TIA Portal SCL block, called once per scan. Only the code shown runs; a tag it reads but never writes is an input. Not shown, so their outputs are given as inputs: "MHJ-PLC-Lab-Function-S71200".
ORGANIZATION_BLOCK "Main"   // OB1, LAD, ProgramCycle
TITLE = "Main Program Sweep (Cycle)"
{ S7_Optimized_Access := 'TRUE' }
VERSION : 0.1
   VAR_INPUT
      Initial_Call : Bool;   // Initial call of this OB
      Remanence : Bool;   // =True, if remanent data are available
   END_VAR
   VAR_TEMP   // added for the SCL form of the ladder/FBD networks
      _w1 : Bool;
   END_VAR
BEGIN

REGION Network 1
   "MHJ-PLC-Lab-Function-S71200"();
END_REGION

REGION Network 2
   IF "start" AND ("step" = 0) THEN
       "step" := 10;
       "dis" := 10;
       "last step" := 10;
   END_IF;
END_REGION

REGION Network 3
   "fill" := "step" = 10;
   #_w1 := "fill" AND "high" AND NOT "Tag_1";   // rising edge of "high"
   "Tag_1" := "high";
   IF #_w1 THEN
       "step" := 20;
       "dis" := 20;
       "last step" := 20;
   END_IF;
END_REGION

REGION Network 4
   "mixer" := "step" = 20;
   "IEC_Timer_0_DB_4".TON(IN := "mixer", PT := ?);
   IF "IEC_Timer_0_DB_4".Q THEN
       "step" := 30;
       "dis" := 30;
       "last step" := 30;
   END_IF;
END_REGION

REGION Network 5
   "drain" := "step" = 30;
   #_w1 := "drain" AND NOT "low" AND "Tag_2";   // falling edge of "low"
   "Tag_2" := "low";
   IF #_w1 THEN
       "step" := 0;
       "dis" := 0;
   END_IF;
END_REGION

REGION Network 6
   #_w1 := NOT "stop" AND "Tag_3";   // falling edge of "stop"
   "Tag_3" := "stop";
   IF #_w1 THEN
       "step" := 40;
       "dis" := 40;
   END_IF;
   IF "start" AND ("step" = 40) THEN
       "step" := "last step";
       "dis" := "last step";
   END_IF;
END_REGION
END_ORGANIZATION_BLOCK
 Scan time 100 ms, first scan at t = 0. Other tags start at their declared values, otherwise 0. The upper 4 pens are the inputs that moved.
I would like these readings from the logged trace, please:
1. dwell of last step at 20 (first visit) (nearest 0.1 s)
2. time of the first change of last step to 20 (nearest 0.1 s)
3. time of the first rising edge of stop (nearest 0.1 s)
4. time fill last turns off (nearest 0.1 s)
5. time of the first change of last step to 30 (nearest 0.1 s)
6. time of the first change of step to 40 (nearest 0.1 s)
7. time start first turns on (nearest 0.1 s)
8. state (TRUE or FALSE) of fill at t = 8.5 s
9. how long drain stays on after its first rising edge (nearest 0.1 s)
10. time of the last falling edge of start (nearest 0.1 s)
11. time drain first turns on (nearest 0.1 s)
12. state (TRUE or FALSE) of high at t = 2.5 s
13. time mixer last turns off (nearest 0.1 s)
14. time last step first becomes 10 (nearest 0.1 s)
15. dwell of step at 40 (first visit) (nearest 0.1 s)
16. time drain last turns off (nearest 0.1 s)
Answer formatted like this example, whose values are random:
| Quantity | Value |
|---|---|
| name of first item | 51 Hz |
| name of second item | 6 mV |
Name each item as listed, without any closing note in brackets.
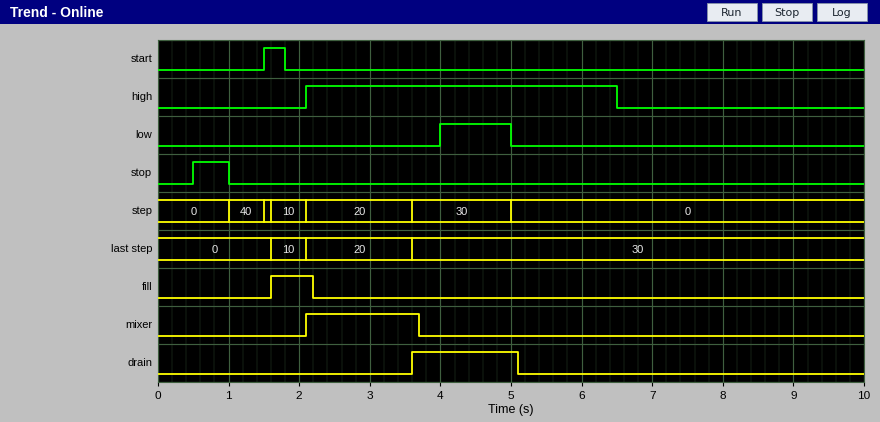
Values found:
| Quantity | Value |
|---|---|
| dwell of last step at 20 (first visit) | 1.5 s |
| time of the first change of last step to 20 | 2.1 s |
| time of the first rising edge of stop | 0.5 s |
| time fill last turns off | 2.2 s |
| time of the first change of last step to 30 | 3.6 s |
| time of the first change of step to 40 | 1.0 s |
| time start first turns on | 1.5 s |
| state (TRUE or FALSE) of fill at t = 8.5 s | FALSE |
| how long drain stays on after its first rising edge | 1.5 s |
| time of the last falling edge of start | 1.8 s |
| time drain first turns on | 3.6 s |
| state (TRUE or FALSE) of high at t = 2.5 s | TRUE |
| time mixer last turns off | 3.7 s |
| time last step first becomes 10 | 1.6 s |
| dwell of step at 40 (first visit) | 0.5 s |
| time drain last turns off | 5.1 s |
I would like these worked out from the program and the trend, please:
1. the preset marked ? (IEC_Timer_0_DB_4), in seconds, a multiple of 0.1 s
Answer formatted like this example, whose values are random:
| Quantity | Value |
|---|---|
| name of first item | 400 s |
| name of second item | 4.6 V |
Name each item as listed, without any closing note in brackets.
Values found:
| Quantity | Value |
|---|---|
| the preset marked ? (IEC_Timer_0_DB_4), in seconds, a multiple of 0.1 s | 1.5 s |
